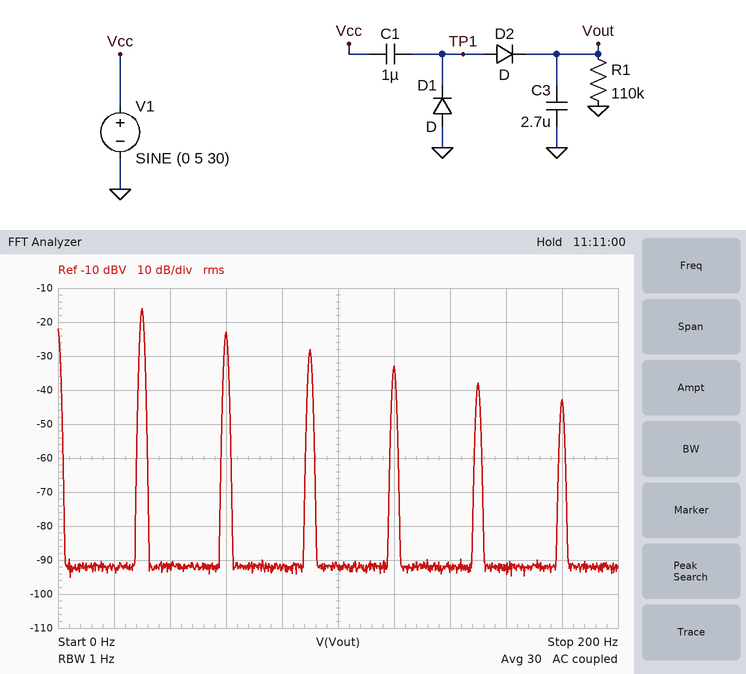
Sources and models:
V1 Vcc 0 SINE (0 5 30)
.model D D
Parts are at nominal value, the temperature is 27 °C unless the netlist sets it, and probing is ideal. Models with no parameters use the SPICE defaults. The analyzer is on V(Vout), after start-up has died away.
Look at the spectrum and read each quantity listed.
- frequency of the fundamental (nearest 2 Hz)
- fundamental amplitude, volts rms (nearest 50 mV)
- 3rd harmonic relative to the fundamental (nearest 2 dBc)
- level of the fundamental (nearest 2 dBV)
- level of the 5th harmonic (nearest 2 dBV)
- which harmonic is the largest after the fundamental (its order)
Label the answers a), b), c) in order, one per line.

a) 30 Hz
b) 150 mV
c) -12 dBc
d) -16 dBV
e) -38 dBV
f) 2
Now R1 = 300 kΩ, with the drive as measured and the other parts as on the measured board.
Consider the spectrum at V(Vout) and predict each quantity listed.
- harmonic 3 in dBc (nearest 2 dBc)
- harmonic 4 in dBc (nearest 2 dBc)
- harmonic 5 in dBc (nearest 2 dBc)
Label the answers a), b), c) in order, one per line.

a) -10 dBc
b) -14 dBc
c) -18 dBc
